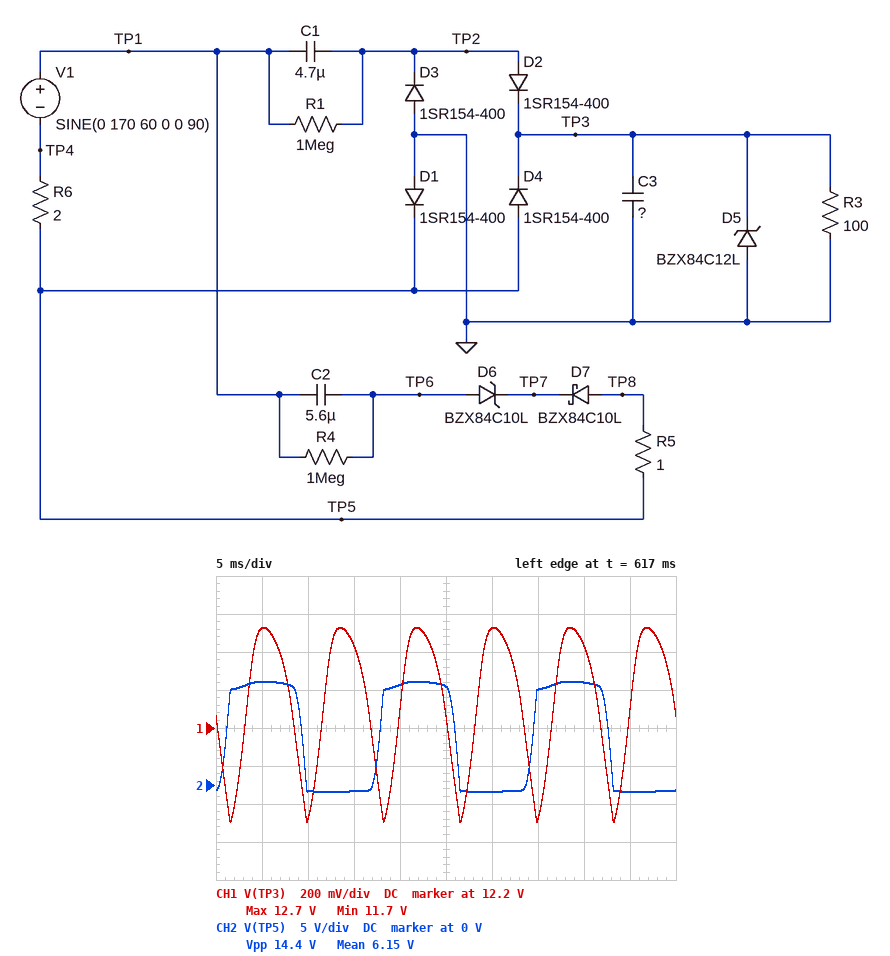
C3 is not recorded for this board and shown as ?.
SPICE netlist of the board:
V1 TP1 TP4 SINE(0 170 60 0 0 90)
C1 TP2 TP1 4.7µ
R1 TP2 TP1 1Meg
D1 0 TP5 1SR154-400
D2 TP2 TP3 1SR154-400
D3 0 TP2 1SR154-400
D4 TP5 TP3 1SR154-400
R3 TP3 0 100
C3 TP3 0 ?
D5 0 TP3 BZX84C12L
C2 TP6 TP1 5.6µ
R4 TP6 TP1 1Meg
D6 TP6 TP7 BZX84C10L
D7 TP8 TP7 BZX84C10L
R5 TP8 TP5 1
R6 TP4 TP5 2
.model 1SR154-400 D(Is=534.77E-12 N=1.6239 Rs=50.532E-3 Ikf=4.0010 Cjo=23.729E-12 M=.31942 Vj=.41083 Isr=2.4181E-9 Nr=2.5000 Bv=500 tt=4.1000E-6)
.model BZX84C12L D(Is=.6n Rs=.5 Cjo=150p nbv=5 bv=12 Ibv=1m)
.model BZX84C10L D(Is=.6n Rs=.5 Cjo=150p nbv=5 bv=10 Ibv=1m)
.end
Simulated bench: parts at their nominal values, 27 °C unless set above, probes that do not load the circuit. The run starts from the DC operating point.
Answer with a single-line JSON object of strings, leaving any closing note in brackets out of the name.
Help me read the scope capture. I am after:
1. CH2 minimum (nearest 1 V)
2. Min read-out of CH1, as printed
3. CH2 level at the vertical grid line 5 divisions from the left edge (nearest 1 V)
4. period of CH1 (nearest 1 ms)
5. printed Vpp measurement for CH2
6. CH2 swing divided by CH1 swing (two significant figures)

{"CH2 minimum": "-1 V", "Min read-out of CH1, as printed": "11.7 V", "CH2 level at the vertical grid line 5 divisions from the left edge": "13 V", "period of CH1": "8 ms", "printed Vpp measurement for CH2": "14.4 V", "CH2 swing divided by CH1 swing": "14"}
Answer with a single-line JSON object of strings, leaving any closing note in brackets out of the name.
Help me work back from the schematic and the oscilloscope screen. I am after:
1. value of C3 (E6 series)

{"value of C3": "330 µF"}
